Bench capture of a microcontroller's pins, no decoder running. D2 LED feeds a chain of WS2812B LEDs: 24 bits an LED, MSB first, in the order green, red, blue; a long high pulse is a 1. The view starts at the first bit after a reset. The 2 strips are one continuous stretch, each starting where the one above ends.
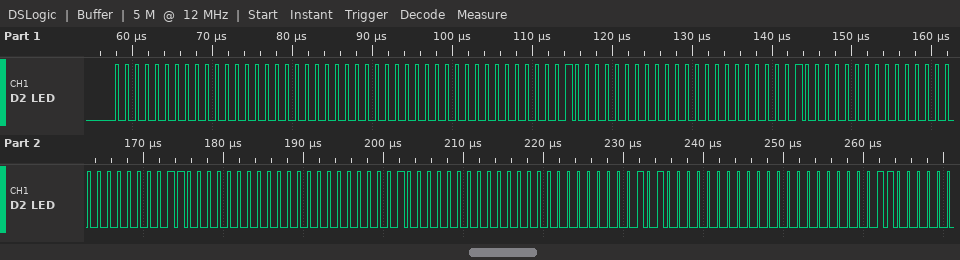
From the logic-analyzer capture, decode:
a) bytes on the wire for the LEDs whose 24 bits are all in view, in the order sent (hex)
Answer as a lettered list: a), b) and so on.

a) 00 00 00 00 00 04 00 00 08 00 00 0C 00 00 10 00 00 14 00 00 18
